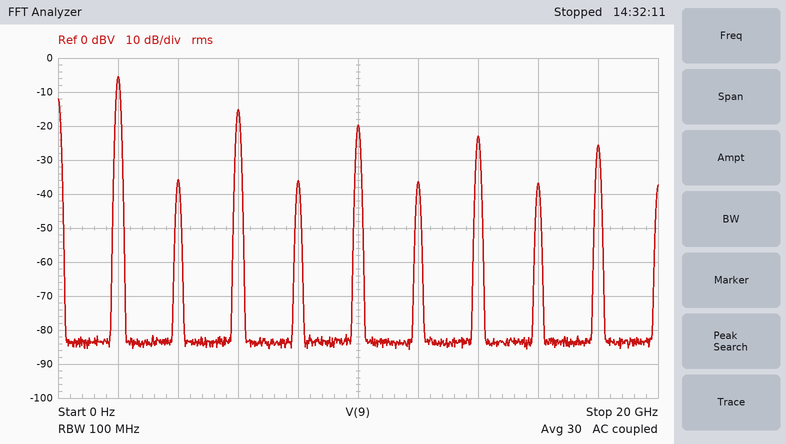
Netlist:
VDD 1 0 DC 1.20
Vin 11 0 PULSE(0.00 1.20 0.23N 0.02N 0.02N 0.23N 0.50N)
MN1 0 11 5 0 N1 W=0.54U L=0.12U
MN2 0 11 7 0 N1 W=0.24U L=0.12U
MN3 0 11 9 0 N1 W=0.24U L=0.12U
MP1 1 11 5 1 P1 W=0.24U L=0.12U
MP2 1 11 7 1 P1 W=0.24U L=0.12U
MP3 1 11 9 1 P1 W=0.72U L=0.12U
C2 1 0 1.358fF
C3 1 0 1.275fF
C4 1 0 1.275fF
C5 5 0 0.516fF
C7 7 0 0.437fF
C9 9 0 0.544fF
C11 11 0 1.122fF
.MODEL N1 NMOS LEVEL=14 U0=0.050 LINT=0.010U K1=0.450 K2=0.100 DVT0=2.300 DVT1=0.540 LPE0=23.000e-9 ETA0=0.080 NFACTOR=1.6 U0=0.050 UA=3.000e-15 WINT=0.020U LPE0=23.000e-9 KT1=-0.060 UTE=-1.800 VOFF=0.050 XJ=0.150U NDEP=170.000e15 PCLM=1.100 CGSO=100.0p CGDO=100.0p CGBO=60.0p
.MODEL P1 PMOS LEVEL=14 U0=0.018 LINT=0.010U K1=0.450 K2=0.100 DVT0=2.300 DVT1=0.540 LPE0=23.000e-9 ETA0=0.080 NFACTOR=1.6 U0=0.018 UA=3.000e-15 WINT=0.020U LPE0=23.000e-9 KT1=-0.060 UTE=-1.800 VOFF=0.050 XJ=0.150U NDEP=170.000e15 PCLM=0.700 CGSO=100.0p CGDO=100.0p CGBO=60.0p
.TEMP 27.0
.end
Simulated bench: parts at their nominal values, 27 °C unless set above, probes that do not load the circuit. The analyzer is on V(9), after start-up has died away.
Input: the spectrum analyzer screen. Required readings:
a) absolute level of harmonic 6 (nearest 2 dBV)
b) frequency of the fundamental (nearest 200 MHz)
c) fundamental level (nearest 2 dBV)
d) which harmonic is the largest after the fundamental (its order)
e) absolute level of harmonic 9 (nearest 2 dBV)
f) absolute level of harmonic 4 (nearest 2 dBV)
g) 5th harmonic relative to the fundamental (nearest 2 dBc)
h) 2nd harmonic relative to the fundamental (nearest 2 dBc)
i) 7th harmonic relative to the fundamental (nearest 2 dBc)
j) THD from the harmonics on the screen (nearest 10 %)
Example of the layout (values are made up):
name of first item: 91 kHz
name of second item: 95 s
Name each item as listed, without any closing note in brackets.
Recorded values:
absolute level of harmonic 6: -36 dBV
frequency of the fundamental: 2.0 GHz
fundamental level: -6 dBV
which harmonic is the largest after the fundamental: 3
absolute level of harmonic 9: -26 dBV
absolute level of harmonic 4: -36 dBV
5th harmonic relative to the fundamental: -14 dBc
2nd harmonic relative to the fundamental: -30 dBc
7th harmonic relative to the fundamental: -18 dBc
THD from the harmonics on the screen: 40 %
